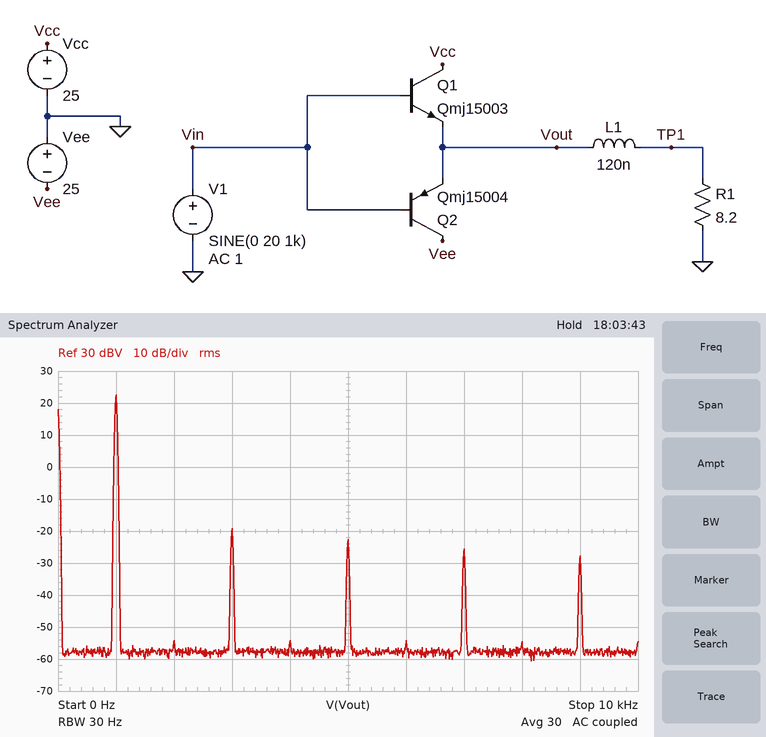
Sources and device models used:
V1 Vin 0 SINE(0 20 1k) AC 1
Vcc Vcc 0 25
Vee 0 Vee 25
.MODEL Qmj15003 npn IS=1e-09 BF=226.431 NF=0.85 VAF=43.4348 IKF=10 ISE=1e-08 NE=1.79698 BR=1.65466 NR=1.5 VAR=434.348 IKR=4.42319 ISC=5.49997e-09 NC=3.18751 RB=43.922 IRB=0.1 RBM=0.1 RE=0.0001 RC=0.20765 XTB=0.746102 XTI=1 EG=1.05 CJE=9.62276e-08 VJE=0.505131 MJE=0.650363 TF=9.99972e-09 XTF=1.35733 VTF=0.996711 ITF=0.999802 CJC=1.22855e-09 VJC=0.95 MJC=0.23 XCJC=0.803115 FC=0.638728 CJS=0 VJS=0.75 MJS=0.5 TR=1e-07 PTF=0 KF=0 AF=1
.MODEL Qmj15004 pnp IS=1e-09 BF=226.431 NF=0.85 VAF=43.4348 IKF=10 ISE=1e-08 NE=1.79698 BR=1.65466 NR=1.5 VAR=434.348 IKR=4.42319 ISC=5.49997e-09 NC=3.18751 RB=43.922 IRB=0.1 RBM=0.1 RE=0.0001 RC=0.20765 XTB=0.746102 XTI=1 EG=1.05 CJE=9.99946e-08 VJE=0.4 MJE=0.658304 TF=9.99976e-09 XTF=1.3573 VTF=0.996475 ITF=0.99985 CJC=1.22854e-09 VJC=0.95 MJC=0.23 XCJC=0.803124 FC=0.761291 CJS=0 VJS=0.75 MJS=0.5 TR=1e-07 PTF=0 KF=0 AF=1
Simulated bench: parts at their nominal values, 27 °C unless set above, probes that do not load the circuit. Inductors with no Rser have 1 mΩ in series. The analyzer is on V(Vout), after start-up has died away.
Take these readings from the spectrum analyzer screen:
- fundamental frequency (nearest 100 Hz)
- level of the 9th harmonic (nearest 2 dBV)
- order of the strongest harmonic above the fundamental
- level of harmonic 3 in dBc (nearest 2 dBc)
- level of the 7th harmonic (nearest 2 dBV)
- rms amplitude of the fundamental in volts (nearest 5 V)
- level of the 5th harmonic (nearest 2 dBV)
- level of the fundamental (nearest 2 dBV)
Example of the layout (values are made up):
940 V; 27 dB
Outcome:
1.0 kHz; -28 dBV; 3; -42 dBc; -26 dBV; 15 V; -22 dBV; 22 dBV
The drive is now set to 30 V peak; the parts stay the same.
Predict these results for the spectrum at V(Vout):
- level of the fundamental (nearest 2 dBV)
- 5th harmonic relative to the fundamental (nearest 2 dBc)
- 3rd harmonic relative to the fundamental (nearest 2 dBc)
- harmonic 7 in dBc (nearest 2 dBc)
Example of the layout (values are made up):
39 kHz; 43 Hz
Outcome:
26 dBV; -30 dBc; -26 dBc; -44 dBc
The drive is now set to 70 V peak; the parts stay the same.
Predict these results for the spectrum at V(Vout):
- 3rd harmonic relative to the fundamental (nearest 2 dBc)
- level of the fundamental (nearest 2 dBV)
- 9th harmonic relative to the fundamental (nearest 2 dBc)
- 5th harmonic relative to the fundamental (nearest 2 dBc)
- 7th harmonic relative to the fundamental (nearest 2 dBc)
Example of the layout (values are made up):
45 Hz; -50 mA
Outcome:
-12 dBc; 28 dBV; -44 dBc; -20 dBc; -32 dBc
